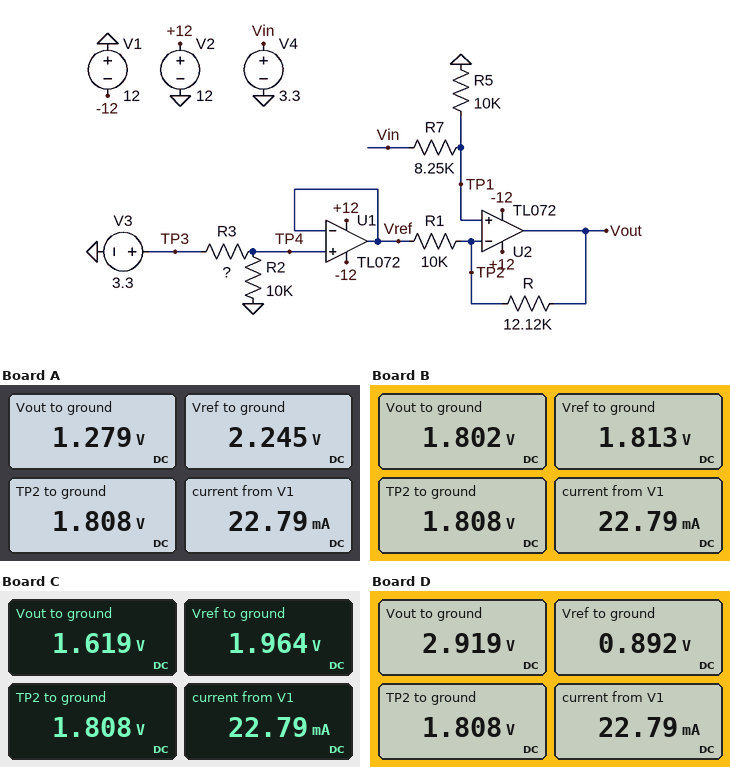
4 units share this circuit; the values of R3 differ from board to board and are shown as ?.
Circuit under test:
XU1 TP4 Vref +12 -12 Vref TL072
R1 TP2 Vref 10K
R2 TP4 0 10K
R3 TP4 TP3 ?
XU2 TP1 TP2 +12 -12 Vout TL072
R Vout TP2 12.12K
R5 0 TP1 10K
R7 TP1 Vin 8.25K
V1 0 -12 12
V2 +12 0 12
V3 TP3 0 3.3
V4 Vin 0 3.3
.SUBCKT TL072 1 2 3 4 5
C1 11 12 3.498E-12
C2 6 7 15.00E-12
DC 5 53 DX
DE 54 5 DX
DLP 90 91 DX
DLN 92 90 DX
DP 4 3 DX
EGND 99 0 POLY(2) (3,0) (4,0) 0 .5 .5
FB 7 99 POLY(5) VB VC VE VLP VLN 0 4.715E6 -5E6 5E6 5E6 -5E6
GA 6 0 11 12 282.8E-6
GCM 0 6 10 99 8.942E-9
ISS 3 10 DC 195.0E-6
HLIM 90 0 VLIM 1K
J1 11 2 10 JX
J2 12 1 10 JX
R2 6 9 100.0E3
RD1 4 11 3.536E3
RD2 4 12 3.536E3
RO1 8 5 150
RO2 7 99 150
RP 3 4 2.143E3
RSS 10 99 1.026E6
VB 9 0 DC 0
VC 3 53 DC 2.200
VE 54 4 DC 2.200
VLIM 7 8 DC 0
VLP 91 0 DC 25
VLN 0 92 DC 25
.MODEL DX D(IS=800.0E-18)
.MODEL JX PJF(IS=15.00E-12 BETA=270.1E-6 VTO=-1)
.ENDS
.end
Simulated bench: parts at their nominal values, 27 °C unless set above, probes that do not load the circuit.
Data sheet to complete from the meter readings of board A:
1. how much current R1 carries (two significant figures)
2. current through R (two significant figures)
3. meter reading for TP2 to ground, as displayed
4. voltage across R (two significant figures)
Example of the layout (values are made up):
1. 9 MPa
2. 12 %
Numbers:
1. 44 µA
2. 44 µA
3. 1.808 V
4. 530 mV
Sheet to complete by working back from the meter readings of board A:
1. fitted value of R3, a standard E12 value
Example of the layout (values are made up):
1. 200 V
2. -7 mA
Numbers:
1. 4.7 kΩ
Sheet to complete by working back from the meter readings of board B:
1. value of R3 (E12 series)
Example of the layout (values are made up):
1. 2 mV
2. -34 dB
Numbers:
1. 8.2 kΩ
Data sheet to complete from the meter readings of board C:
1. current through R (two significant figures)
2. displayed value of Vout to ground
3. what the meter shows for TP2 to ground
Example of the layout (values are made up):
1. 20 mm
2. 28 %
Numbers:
1. 16 µA
2. 1.619 V
3. 1.808 V
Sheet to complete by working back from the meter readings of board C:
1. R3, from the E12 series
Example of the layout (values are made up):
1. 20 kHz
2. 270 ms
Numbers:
1. 6.8 kΩ
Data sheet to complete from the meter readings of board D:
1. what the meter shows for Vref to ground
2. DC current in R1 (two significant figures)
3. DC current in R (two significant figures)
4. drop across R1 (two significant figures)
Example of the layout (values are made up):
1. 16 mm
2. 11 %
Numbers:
1. 0.892 V
2. 92 µA
3. 92 µA
4. 920 mV
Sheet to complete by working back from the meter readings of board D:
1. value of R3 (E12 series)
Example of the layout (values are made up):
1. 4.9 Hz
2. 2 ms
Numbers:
1. 27 kΩ
